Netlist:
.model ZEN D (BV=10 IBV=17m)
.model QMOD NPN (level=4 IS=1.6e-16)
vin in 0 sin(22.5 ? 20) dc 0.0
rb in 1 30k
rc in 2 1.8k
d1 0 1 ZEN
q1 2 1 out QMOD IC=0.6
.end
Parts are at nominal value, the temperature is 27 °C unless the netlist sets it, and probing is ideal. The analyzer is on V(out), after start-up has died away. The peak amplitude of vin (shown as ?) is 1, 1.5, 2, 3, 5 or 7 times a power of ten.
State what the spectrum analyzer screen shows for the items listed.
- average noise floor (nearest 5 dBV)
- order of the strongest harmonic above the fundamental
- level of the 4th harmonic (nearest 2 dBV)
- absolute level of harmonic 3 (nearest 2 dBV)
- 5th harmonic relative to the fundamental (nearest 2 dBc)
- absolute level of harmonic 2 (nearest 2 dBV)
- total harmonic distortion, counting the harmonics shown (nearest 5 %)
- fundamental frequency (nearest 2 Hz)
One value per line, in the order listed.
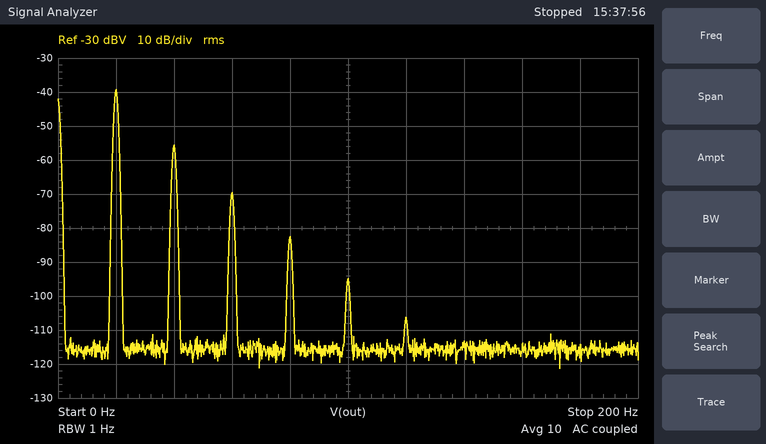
-115 dBV
2
-82 dBV
-70 dBV
-56 dBc
-56 dBV
15 %
20 Hz
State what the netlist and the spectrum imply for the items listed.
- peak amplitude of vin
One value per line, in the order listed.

7 V
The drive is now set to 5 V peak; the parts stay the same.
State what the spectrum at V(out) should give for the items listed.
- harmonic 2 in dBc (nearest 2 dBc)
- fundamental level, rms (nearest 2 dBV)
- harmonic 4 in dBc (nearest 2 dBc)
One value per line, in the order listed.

-20 dBc
-42 dBV
-54 dBc
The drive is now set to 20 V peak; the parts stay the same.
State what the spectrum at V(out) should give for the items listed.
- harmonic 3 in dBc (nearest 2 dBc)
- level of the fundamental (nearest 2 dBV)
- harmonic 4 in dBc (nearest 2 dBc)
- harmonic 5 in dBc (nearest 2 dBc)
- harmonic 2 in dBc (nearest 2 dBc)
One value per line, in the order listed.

-6 dBc
6 dBV
-14 dBc
-34 dBc
-2 dBc
